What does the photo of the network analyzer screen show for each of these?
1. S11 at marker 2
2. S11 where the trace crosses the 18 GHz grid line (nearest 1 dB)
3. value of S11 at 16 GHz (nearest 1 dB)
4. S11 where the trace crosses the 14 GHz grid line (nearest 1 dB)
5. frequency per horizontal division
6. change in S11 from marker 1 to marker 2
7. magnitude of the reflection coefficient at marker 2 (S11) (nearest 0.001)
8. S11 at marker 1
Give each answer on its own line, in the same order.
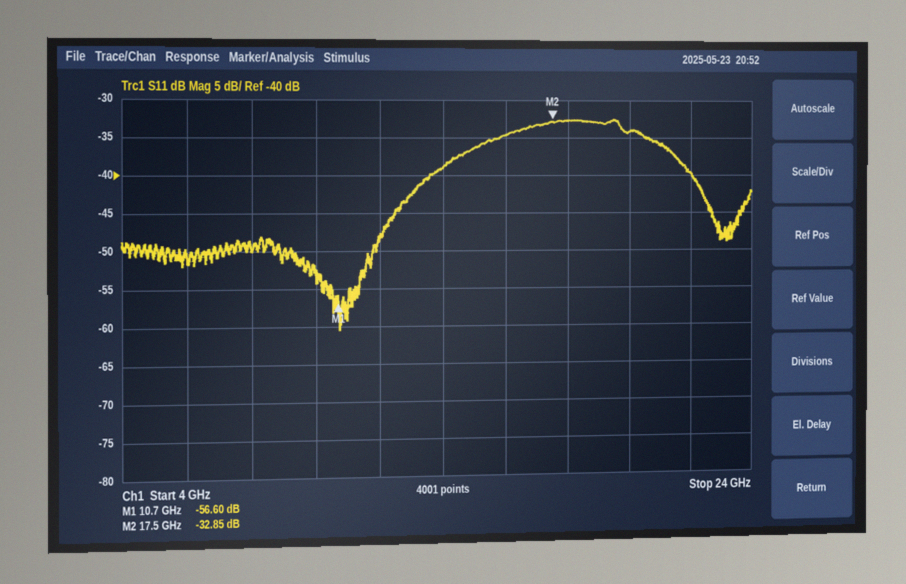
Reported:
-32.85 dB
-33 dB
-35 dB
-39 dB
2 GHz
23.75 dB
0.023
-56.60 dB
